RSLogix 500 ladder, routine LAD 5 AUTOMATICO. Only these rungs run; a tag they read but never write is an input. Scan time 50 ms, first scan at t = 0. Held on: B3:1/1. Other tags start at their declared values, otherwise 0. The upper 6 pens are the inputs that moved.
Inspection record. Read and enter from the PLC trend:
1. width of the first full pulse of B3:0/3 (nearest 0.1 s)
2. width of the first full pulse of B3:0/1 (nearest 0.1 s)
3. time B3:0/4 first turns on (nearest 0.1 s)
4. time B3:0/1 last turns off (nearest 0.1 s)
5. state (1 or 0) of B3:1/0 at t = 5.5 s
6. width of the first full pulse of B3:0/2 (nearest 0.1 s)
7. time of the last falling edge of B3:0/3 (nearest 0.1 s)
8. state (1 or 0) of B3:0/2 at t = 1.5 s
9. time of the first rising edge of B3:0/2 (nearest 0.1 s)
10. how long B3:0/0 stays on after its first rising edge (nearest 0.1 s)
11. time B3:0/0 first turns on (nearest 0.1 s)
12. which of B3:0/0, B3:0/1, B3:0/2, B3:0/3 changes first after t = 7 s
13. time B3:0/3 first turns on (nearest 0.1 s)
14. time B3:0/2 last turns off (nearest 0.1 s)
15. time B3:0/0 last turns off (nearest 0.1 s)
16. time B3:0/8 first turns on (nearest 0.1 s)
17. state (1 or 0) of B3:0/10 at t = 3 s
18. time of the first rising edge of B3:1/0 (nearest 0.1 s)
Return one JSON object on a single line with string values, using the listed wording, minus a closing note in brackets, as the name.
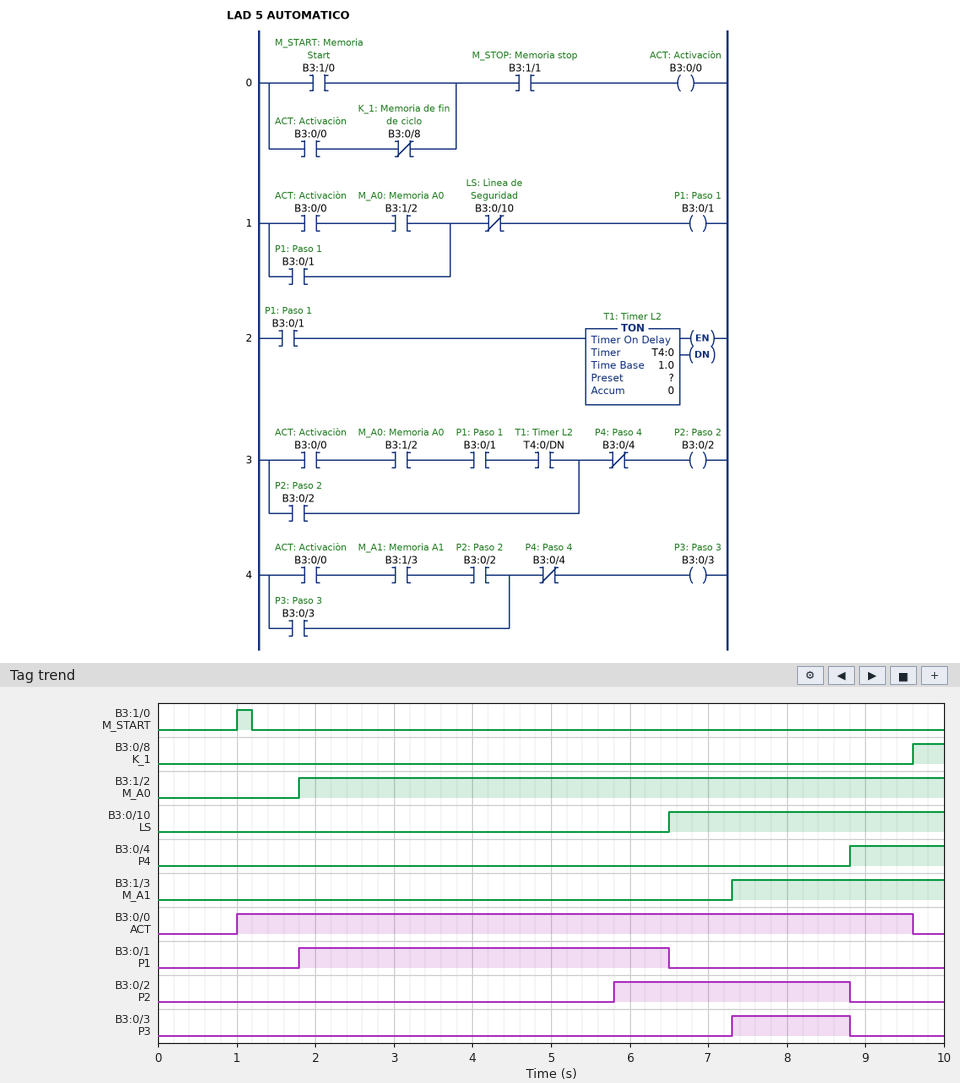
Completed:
{"width of the first full pulse of B3:0/3": "1.5 s", "width of the first full pulse of B3:0/1": "4.7 s", "time B3:0/4 first turns on": "8.8 s", "time B3:0/1 last turns off": "6.5 s", "state (1 or 0) of B3:1/0 at t = 5.5 s": "0", "width of the first full pulse of B3:0/2": "3.0 s", "time of the last falling edge of B3:0/3": "8.8 s", "state (1 or 0) of B3:0/2 at t = 1.5 s": "0", "time of the first rising edge of B3:0/2": "5.8 s", "how long B3:0/0 stays on after its first rising edge": "8.6 s", "time B3:0/0 first turns on": "1.0 s", "which of B3:0/0, B3:0/1, B3:0/2, B3:0/3 changes first after t = 7 s": "B3:0/3", "time B3:0/3 first turns on": "7.3 s", "time B3:0/2 last turns off": "8.8 s", "time B3:0/0 last turns off": "9.6 s", "time B3:0/8 first turns on": "9.6 s", "state (1 or 0) of B3:0/10 at t = 3 s": "0", "time of the first rising edge of B3:1/0": "1.0 s"}
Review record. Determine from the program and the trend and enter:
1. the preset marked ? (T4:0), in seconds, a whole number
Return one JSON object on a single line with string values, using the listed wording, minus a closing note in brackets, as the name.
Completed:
{"the preset marked ? (T4:0), in seconds, a whole number": "4 s"}
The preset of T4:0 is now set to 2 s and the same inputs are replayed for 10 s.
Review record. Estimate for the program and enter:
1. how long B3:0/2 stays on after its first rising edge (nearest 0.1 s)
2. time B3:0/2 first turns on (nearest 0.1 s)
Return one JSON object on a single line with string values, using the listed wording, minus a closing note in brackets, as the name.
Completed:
{"how long B3:0/2 stays on after its first rising edge": "5.0 s", "time B3:0/2 first turns on": "3.8 s"}
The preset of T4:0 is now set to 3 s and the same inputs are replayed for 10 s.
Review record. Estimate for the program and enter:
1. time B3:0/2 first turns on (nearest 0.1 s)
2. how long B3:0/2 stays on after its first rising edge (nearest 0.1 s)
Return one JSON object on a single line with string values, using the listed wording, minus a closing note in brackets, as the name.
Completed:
{"time B3:0/2 first turns on": "4.8 s", "how long B3:0/2 stays on after its first rising edge": "4.0 s"}
